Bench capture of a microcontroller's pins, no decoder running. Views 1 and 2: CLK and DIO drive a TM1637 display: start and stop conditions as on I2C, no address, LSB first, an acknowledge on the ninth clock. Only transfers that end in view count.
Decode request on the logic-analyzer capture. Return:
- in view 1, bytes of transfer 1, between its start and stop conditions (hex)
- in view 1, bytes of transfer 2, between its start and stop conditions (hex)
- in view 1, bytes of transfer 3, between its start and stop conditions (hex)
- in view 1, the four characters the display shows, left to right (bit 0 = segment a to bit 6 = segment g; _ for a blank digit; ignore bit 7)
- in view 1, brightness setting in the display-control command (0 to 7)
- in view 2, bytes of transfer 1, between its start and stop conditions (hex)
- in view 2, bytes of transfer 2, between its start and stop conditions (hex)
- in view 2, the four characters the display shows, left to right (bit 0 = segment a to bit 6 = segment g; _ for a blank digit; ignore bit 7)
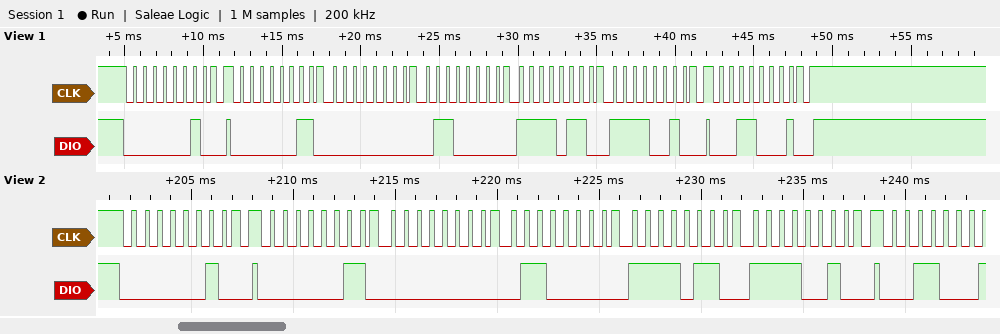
40
C0 00 06 6F 4F
8C
_193
4
40
C0 00 06 6F 4F
_193
